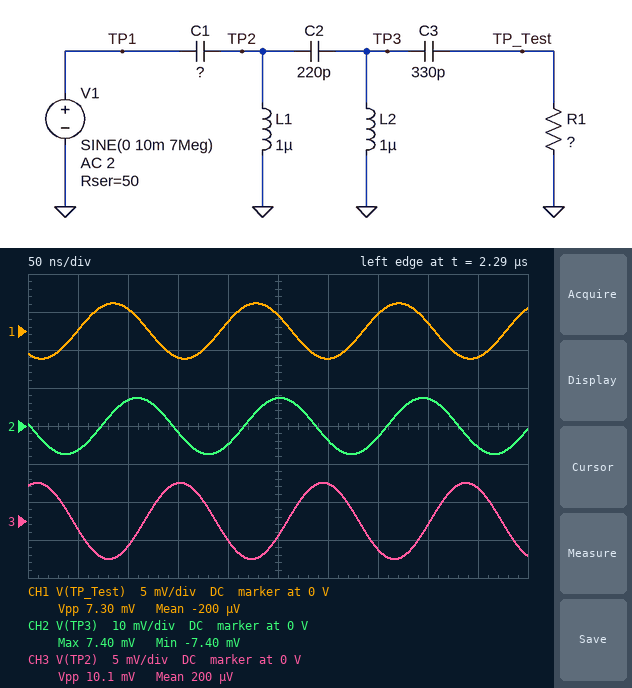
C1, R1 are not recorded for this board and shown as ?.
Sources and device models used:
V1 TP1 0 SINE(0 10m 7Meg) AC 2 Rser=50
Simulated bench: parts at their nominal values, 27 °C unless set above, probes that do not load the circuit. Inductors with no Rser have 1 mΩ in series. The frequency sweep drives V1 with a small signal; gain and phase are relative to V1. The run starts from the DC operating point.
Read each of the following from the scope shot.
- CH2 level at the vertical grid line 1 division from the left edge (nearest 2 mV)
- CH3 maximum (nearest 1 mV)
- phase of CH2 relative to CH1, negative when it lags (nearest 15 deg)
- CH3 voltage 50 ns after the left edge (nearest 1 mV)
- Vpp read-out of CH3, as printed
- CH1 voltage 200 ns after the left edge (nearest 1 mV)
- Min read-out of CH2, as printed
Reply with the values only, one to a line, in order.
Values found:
-6 mV
5 mV
-60 deg
-1 mV
10.1 mV
1 mV
-7.40 mV
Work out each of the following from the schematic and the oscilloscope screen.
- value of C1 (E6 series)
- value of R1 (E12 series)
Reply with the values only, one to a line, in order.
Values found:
220 pF
39 Ω
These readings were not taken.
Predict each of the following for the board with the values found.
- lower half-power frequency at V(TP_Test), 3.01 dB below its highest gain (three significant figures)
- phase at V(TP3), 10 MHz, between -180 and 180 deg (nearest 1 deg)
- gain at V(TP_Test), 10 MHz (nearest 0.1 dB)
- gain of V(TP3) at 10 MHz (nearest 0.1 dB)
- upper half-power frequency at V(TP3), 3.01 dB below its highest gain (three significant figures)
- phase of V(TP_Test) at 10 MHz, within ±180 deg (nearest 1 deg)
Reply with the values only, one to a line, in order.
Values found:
5.90 MHz
107 deg
-7.3 dB
-3.3 dB
11.7 MHz
158 deg
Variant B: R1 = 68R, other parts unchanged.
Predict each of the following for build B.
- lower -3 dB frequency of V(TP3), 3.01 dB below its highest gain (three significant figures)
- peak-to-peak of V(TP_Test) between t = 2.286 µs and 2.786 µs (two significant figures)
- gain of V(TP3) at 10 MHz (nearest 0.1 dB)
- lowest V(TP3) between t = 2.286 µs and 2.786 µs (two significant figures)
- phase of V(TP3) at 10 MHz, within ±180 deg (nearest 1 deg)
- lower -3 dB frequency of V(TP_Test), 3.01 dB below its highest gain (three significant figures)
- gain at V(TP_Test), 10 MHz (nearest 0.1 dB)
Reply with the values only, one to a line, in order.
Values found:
5.98 MHz
11 mV
-3.7 dB
-7.7 mV
120 deg
6.05 MHz
-5.5 dB
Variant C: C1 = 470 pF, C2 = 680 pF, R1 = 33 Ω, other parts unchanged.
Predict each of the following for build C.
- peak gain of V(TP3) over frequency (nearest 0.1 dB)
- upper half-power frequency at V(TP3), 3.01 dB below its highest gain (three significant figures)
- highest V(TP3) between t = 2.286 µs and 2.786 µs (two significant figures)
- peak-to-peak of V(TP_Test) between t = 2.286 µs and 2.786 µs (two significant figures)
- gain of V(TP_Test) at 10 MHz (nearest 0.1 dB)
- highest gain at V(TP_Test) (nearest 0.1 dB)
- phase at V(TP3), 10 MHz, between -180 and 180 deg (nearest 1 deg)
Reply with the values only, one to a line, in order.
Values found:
3.0 dB
4.10 MHz
6.3 mV
5.4 mV
-8.2 dB
-7.9 dB
62 deg
